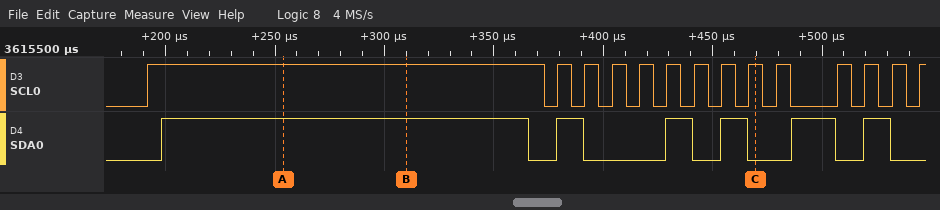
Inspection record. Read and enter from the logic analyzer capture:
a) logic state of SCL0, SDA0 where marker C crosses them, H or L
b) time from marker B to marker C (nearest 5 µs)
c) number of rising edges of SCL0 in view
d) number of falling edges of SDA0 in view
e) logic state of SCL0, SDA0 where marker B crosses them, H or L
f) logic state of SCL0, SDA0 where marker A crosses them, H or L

SCL0=H, SDA0=L
160 µs
14
6
SCL0=H, SDA0=H
SCL0=H, SDA0=H
